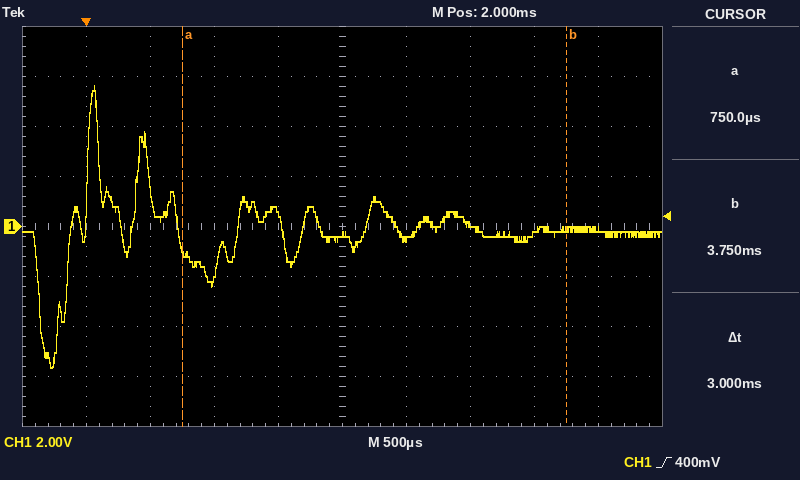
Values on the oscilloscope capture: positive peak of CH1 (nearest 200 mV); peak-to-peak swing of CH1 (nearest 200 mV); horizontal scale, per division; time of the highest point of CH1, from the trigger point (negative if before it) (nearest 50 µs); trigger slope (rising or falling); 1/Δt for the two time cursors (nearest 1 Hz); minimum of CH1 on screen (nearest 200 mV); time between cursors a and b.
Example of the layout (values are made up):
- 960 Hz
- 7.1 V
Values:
- 5.6 V
- 11.2 V
- 500 µs
- +50 µs
- rising
- 333 Hz
- -5.6 V
- 3 ms
